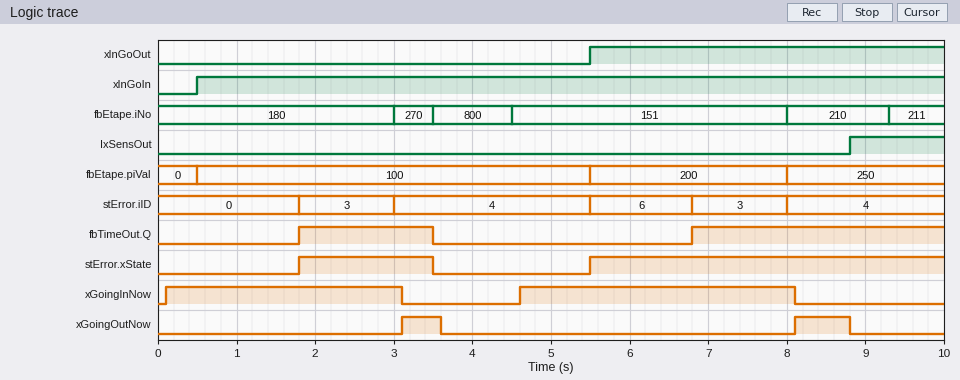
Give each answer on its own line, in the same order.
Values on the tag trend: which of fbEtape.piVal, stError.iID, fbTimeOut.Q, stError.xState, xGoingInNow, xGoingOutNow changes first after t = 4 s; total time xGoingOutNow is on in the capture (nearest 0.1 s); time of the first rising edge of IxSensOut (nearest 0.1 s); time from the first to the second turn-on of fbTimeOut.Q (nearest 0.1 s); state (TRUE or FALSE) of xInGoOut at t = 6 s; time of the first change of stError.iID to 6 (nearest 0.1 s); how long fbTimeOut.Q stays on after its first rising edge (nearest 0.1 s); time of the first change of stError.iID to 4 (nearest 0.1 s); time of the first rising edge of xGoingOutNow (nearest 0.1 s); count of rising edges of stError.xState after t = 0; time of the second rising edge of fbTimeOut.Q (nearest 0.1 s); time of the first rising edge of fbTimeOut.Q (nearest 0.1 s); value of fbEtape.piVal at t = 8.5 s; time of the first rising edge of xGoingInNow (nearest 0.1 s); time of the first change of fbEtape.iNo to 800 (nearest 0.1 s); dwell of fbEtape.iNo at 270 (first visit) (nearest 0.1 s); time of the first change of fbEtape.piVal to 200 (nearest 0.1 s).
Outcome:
xGoingInNow
1.2 s
8.8 s
5.0 s
TRUE
5.5 s
1.7 s
3.0 s
3.1 s
2
6.8 s
1.8 s
250
0.1 s
3.5 s
0.5 s
5.5 s
